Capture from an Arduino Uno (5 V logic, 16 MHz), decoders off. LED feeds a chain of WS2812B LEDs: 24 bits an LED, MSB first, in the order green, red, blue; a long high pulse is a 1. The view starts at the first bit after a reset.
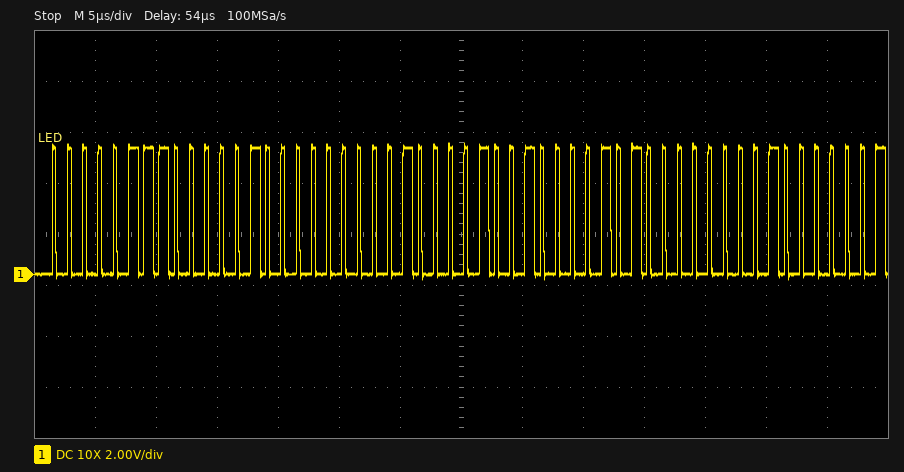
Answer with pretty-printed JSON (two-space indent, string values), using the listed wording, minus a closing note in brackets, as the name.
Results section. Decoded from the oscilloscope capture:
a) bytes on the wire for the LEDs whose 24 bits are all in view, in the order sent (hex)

{
  "bytes on the wire for the LEDs whose 24 bits are all in view, in the order sent": "07 04 01 09 0A 01"
}
